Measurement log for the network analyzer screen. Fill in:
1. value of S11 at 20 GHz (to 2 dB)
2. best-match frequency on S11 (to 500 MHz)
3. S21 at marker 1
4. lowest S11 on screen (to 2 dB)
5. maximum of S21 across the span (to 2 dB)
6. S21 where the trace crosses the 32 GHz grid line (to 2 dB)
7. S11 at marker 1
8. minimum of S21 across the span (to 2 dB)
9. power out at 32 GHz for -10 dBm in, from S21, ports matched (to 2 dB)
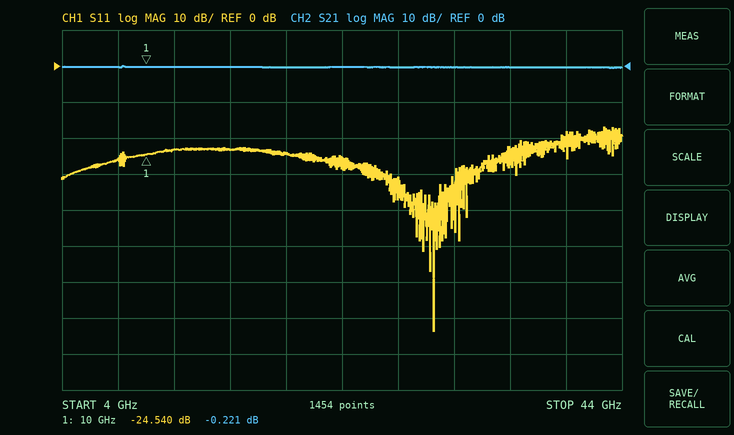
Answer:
-24 dB
30.5 GHz
-0.221 dB
-74 dB
0 dB
0 dB
-24.540 dB
0 dB
-10 dBm
